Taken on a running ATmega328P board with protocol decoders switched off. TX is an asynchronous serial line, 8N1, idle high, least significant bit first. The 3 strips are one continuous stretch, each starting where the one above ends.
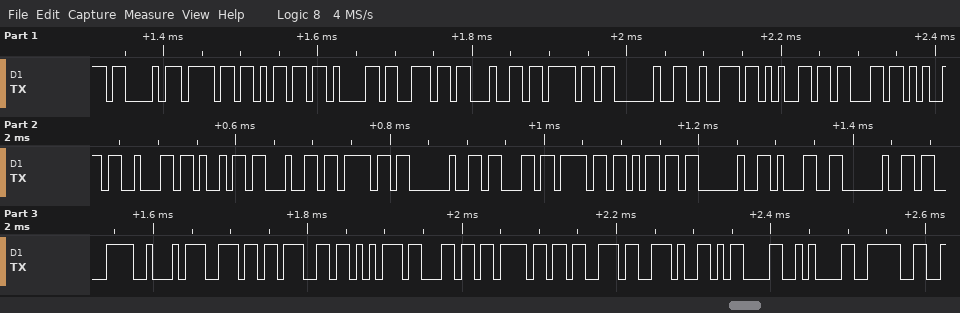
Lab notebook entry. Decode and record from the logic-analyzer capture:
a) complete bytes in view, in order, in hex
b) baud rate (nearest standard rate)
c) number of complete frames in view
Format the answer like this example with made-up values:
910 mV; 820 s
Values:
43 6F 6D 61 6E 64 6F 20 72 65 63 65 62 69 64 6F 20 63 6F 6D 20 31 20 C3 A2 6E 67 75 6C 6F 73 2E 0D 0A 3E; 115200 baud; 35
